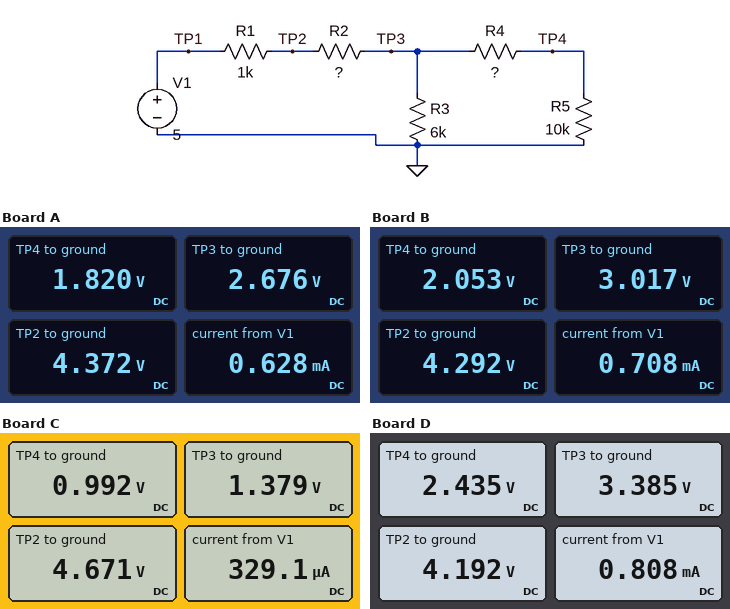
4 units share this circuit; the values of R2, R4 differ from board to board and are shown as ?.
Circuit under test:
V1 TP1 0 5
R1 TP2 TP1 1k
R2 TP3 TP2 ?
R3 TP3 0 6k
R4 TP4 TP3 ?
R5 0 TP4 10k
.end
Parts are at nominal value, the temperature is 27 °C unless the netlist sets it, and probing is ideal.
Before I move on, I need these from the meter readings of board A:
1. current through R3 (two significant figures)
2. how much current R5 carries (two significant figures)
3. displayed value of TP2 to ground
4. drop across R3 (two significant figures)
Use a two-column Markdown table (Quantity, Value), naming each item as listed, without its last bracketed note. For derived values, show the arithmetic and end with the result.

| Quantity | Value |
|---|---|
| current through R3 | (2.676 V) / 6 kΩ = 450 µA |
| how much current R5 carries | (1.82 V) / 10 kΩ = 180 µA |
| displayed value of TP2 to ground | 4.372 V |
| drop across R3 | 2.676 V = 2.7 V |
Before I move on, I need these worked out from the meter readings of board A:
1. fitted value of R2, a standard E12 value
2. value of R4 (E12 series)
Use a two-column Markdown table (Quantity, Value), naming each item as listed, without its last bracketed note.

| Quantity | Value |
|---|---|
| fitted value of R2, a standard E12 value | 2.7 kΩ |
| value of R4 | 4.7 kΩ |
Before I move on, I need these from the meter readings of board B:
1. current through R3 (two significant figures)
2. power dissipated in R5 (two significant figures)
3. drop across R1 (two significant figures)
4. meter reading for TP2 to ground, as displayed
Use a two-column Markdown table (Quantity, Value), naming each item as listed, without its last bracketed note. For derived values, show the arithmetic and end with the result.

| Quantity | Value |
|---|---|
| current through R3 | (3.017 V) / 6 kΩ = 500 µA |
| power dissipated in R5 | (2.053 V)^2 / 10 kΩ = 420 µW |
| drop across R1 | 5 V - 4.292 V = 710 mV |
| meter reading for TP2 to ground, as displayed | 4.292 V |
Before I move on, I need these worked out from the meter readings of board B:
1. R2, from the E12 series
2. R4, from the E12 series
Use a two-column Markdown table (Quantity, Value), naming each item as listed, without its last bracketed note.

| Quantity | Value |
|---|---|
| R2, from the E12 series | 1.8 kΩ |
| R4, from the E12 series | 4.7 kΩ |
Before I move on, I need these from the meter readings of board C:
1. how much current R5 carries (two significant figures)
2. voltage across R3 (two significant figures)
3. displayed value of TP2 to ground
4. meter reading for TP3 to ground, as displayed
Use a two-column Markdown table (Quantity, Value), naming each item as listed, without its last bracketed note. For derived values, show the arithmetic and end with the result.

| Quantity | Value |
|---|---|
| how much current R5 carries | (992 mV) / 10 kΩ = 99 µA |
| voltage across R3 | 1.379 V = 1.4 V |
| displayed value of TP2 to ground | 4.671 V |
| meter reading for TP3 to ground, as displayed | 1.379 V |
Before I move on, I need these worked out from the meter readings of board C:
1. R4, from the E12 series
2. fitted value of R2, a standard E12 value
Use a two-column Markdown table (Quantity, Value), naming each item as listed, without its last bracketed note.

| Quantity | Value |
|---|---|
| R4, from the E12 series | 3.9 kΩ |
| fitted value of R2, a standard E12 value | 10 kΩ |
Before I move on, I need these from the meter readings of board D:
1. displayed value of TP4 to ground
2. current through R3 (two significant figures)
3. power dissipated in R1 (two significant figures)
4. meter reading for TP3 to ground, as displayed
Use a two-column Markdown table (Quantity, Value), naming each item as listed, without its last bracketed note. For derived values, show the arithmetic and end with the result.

| Quantity | Value |
|---|---|
| displayed value of TP4 to ground | 2.435 V |
| current through R3 | (3.385 V) / 6 kΩ = 560 µA |
| power dissipated in R1 | (5 V - 4.192 V)^2 / 1 kΩ = 650 µW |
| meter reading for TP3 to ground, as displayed | 3.385 V |
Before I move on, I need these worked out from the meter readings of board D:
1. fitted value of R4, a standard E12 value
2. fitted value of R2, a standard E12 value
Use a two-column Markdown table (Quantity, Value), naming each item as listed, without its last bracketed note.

| Quantity | Value |
|---|---|
| fitted value of R4, a standard E12 value | 3.9 kΩ |
| fitted value of R2, a standard E12 value | 1 kΩ |
